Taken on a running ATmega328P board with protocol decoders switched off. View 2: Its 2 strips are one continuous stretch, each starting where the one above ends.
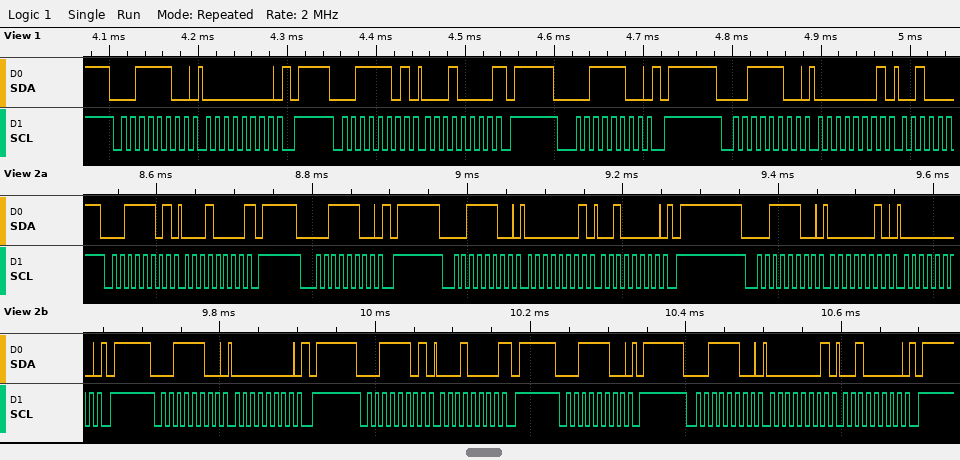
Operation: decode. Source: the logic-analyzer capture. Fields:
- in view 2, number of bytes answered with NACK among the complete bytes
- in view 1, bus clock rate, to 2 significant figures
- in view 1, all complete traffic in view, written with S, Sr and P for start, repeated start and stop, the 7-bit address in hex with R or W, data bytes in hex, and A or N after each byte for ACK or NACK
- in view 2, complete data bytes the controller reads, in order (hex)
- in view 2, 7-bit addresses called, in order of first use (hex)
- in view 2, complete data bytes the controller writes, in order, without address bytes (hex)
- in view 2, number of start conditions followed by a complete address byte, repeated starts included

2
100 kHz
S 1EW A 00 A P S 1ER A 10 N P S 1EW A P S 1EW A 01 A
10 10
0x1E
01 20 02 00 00 01 20
8
